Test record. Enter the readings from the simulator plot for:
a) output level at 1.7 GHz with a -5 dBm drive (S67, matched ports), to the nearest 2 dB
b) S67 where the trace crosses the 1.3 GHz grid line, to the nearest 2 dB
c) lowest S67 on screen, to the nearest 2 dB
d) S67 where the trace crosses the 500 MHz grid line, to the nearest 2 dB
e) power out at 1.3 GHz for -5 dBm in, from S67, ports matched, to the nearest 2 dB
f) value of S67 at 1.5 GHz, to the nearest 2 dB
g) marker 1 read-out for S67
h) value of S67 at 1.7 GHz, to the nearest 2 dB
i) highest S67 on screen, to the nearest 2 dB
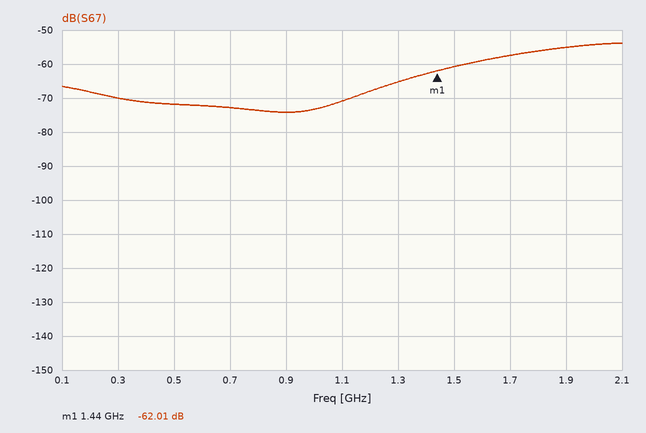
-62 dBm
-66 dB
-74 dB
-72 dB
-70 dBm
-60 dB
-62.01 dB
-58 dB
-54 dB
